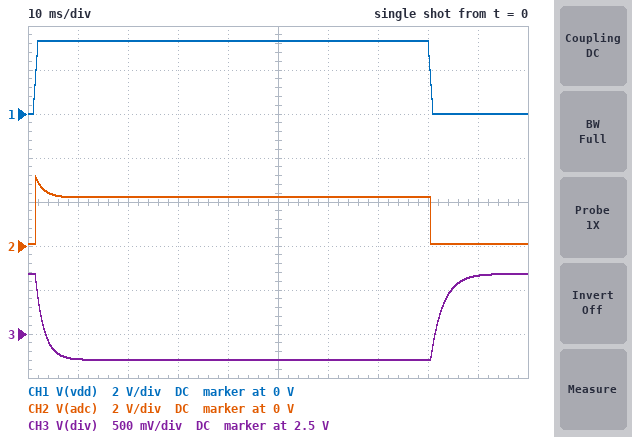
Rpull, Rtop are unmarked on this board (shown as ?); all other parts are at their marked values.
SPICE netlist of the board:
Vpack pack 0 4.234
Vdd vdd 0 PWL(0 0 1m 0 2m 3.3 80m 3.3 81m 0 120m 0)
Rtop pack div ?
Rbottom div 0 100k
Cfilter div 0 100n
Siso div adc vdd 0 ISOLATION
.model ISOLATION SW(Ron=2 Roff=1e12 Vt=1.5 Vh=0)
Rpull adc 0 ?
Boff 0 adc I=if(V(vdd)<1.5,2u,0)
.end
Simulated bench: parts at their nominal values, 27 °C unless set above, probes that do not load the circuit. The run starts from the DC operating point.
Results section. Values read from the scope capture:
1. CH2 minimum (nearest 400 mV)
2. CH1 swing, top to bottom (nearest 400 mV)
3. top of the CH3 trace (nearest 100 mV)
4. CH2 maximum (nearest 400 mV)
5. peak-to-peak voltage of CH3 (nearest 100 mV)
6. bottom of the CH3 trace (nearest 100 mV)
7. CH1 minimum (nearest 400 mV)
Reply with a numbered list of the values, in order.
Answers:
1. 0 V
2. 3.2 V
3. 3.2 V
4. 3.2 V
5. 1.0 V
6. 2.2 V
7. 0 V
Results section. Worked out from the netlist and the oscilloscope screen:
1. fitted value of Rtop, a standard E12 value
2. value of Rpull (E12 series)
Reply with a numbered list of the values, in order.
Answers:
1. 33 kΩ
2. 56 kΩ
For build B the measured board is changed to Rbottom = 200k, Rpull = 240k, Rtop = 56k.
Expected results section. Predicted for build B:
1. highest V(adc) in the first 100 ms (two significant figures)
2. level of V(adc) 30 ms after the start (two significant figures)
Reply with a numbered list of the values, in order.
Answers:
1. 3.3 V
2. 2.8 V
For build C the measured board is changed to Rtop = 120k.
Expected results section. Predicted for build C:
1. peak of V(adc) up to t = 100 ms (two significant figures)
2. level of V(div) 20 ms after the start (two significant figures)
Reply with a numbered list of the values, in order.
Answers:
1. 1.9 V
2. 980 mV
